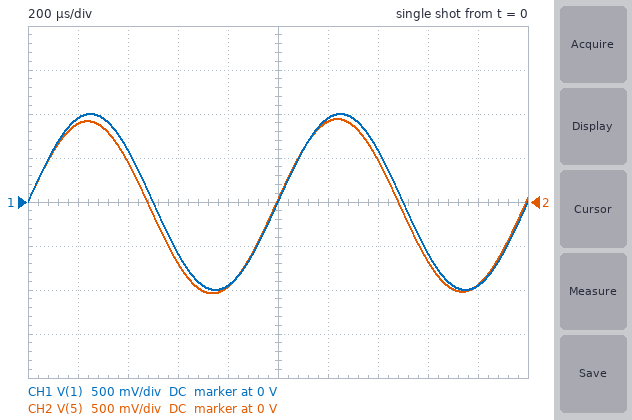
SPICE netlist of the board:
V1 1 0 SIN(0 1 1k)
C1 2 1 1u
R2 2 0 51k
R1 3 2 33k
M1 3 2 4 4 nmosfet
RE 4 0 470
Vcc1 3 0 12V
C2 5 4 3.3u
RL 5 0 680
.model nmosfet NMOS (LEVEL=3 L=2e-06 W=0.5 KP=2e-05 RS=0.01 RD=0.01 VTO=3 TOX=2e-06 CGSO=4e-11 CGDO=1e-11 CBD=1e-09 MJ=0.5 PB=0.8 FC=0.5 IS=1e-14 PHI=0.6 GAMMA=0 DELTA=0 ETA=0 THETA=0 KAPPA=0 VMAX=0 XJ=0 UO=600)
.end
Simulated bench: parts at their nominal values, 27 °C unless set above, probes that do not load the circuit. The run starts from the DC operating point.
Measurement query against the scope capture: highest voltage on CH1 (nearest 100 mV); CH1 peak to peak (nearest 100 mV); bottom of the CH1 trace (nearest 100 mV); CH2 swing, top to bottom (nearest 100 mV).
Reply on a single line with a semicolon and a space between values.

1.0 V; 2.0 V; -1.0 V; 2.0 V
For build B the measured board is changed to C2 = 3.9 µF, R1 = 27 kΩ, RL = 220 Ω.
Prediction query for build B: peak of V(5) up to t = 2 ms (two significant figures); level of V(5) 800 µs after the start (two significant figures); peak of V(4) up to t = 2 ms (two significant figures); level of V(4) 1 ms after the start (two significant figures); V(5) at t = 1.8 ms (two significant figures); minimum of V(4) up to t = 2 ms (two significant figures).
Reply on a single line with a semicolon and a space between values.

920 mV; -910 mV; 5.8 V; 4.8 V; -860 mV; 3.8 V
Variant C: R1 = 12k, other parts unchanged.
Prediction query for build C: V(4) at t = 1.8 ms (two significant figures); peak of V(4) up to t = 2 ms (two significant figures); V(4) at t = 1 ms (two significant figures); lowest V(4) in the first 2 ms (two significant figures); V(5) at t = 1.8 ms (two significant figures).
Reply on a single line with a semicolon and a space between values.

5.7 V; 7.6 V; 6.6 V; 5.6 V; -950 mV
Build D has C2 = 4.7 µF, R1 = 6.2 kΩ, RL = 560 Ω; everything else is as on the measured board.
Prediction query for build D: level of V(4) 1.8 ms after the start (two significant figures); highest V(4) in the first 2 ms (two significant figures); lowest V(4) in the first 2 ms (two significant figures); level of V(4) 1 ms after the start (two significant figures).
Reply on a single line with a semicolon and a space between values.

6.7 V; 8.6 V; 6.6 V; 7.6 V
